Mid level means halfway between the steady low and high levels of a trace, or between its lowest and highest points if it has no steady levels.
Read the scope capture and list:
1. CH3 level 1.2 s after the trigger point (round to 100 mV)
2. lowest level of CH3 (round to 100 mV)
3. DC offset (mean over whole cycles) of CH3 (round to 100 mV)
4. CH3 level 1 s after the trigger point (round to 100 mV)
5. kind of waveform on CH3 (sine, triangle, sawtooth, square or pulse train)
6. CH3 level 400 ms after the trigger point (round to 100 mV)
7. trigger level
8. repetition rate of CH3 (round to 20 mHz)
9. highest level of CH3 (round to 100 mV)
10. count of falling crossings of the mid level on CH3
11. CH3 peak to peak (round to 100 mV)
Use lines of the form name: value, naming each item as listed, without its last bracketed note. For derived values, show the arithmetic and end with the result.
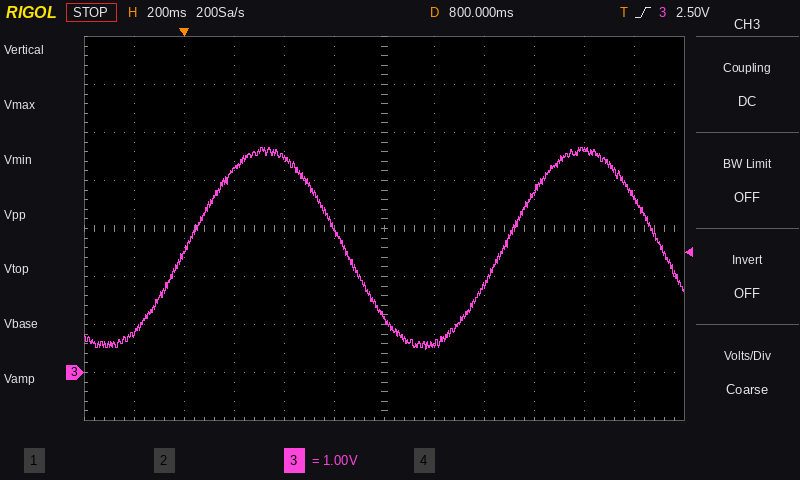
CH3 level 1.2 s after the trigger point: 1.8 V
lowest level of CH3: 500 mV
DC offset (mean over whole cycles) of CH3: (4.7 V + (500 mV)) / 2 ≈ 2.6 V
CH3 level 1 s after the trigger point: 600 mV
kind of waveform on CH3: sine
CH3 level 400 ms after the trigger point: 4.5 V
trigger level: 2.50 V
repetition rate of CH3: 780 mHz
highest level of CH3: 4.7 V
count of falling crossings of the mid level on CH3: 2
CH3 peak to peak: 4.7 V − (500 mV) = 4.2 V
